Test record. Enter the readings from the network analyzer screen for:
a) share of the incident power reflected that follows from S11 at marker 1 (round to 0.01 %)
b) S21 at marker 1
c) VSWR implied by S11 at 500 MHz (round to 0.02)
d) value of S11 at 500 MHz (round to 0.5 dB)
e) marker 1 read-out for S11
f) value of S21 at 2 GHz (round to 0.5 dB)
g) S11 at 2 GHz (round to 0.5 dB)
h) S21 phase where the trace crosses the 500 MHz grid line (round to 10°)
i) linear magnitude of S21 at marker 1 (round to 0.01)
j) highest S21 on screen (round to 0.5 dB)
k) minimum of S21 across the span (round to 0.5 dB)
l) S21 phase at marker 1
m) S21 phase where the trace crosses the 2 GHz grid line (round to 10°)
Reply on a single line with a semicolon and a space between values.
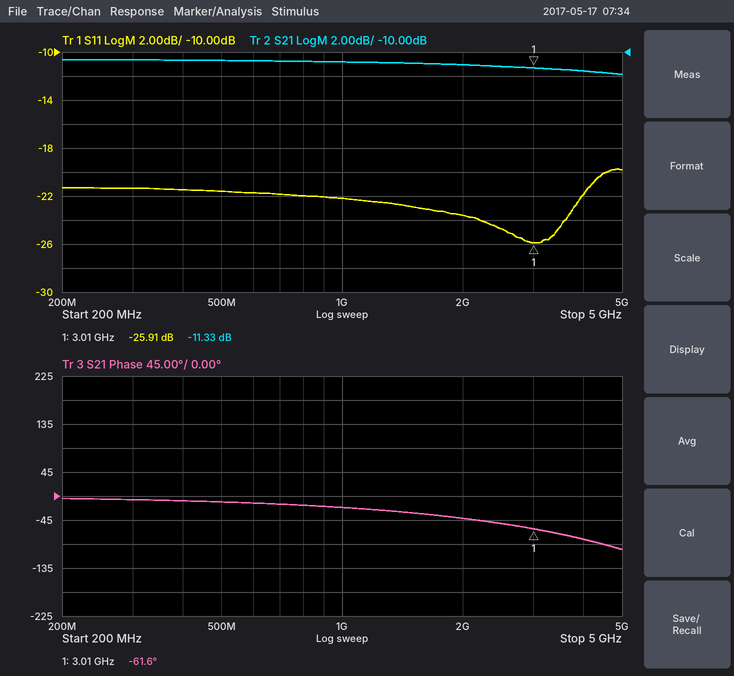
0.26 %; -11.33 dB; 1.18; -21.5 dB; -25.91 dB; -11.0 dB; -23.5 dB; -10°; 0.27; -10.5 dB; -12.0 dB; -61.6°; -40°
